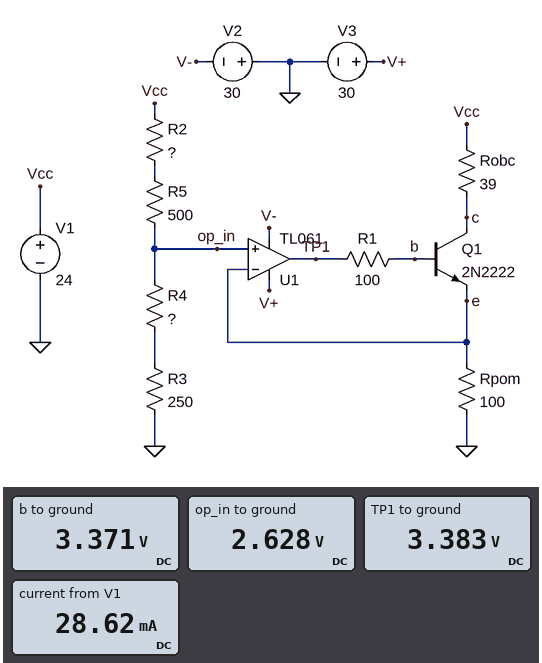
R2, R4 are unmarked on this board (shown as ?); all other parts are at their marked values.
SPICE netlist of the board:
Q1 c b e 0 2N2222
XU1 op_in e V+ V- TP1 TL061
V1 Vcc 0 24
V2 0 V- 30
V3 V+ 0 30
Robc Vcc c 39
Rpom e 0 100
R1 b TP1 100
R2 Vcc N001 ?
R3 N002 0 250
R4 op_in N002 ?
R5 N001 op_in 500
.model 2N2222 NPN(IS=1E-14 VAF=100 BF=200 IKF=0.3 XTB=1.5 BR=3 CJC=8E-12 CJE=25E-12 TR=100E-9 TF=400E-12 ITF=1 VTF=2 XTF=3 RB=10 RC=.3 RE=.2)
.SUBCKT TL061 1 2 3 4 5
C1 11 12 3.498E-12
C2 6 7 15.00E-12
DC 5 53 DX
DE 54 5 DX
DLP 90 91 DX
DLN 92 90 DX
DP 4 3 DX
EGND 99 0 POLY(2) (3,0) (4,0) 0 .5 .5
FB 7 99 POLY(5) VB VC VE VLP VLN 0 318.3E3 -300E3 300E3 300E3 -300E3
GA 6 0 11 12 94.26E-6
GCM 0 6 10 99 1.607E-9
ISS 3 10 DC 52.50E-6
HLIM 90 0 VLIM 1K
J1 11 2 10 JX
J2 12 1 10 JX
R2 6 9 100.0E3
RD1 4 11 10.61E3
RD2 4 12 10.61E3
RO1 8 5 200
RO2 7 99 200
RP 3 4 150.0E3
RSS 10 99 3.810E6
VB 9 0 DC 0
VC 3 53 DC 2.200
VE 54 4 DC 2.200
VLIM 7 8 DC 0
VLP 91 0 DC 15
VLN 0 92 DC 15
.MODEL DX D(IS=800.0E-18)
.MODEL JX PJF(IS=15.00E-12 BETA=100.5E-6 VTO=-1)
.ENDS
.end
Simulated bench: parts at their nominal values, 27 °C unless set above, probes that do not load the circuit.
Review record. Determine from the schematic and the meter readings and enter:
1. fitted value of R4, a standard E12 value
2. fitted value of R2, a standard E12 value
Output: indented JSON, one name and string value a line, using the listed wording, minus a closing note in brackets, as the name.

{
  "fitted value of R4, a standard E12 value": "820 Ω",
  "fitted value of R2, a standard E12 value": "8.2 kΩ"
}
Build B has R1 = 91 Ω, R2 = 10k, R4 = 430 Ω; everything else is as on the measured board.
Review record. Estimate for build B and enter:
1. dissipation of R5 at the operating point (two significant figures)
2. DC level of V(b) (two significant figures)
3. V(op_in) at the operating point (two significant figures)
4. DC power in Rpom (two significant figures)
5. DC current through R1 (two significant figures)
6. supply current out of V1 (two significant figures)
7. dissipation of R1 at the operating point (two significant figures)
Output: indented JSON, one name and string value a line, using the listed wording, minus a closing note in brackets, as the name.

{
  "dissipation of R5 at the operating point": "2.3 mW",
  "DC level of V(b)": "2.2 V",
  "V(op_in) at the operating point": "1.5 V",
  "DC power in Rpom": "21 mW",
  "DC current through R1": "62 µA",
  "supply current out of V1": "17 mA",
  "dissipation of R1 at the operating point": "350 nW"
}
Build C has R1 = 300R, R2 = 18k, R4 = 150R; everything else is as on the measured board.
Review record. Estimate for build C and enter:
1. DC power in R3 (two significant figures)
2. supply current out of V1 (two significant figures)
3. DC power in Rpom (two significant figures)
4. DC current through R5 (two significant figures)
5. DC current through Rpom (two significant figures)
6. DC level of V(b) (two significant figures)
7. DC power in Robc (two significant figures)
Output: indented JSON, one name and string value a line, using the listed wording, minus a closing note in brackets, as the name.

{
  "DC power in R3": "400 µW",
  "supply current out of V1": "6.3 mA",
  "DC power in Rpom": "2.6 mW",
  "DC current through R5": "1.3 mA",
  "DC current through Rpom": "5.1 mA",
  "DC level of V(b)": "1.2 V",
  "DC power in Robc": "1.0 mW"
}
